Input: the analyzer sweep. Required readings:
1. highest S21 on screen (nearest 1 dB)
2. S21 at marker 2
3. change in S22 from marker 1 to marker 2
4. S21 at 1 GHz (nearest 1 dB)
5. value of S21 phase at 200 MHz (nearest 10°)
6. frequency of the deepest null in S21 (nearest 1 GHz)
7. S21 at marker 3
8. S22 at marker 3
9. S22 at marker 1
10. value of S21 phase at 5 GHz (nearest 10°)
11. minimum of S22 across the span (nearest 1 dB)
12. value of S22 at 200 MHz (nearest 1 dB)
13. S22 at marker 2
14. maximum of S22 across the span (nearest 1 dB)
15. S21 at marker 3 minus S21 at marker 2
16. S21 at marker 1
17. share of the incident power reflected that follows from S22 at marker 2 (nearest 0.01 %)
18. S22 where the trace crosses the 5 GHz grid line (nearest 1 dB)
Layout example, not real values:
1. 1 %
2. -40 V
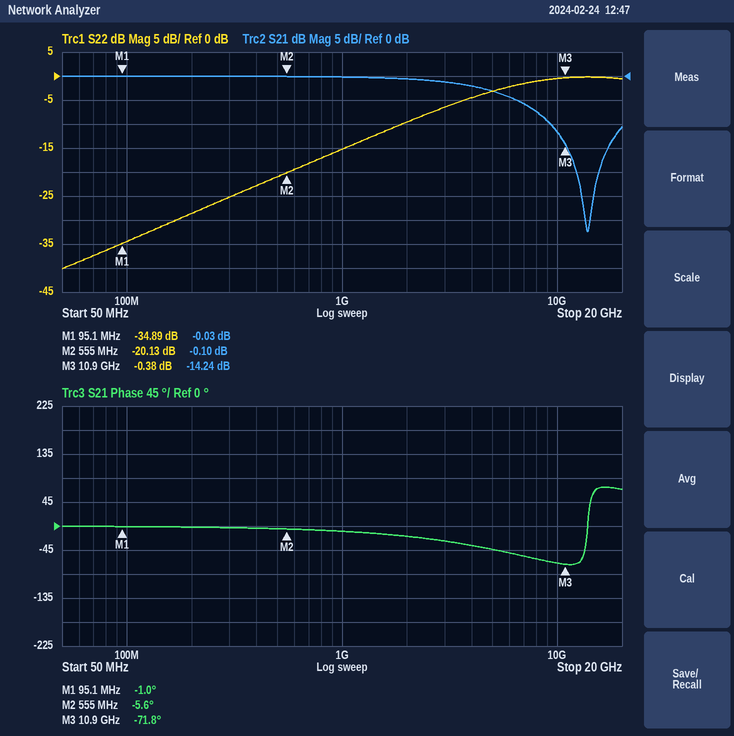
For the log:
1. 0 dB
2. -0.10 dB
3. 14.76 dB
4. 0 dB
5. 0°
6. 14 GHz
7. -14.24 dB
8. -0.38 dB
9. -34.89 dB
10. -40°
11. -40 dB
12. -29 dB
13. -20.13 dB
14. 0 dB
15. -14.14 dB
16. -0.03 dB
17. 0.97 %
18. -3 dB
